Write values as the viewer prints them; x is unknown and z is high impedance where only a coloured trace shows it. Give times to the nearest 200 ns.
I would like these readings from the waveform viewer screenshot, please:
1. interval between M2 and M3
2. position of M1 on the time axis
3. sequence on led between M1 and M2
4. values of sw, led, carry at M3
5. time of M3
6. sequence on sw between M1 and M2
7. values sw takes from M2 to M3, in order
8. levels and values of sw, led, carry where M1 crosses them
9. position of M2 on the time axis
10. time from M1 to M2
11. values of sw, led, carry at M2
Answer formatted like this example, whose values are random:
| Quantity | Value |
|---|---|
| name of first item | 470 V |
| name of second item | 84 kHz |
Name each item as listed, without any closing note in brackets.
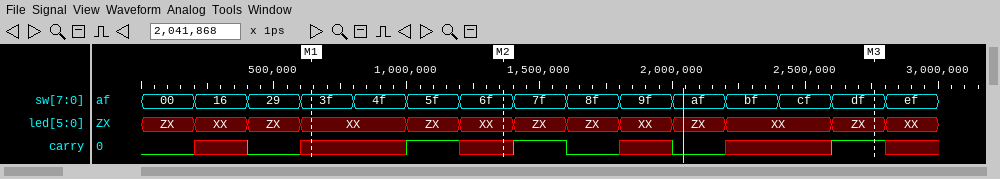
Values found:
| Quantity | Value |
|---|---|
| interval between M2 and M3 | 1400 ns |
| position of M1 on the time axis | 600 ns |
| sequence on led between M1 and M2 | XX, ZX, XX |
| values of sw, led, carry at M3 | sw=df, led=ZX, carry=1 |
| time of M3 | 2800 ns |
| sequence on sw between M1 and M2 | 3f, 4f, 5f, 6f |
| values sw takes from M2 to M3, in order | 6f, 7f, 8f, 9f, af, bf, cf, df |
| levels and values of sw, led, carry where M1 crosses them | sw=3f, led=XX, carry=x |
| position of M2 on the time axis | 1400 ns |
| time from M1 to M2 | 800 ns |
| values of sw, led, carry at M2 | sw=6f, led=XX, carry=x |
